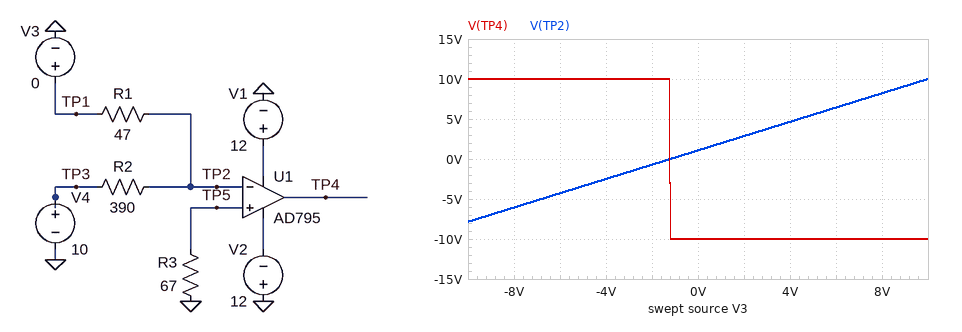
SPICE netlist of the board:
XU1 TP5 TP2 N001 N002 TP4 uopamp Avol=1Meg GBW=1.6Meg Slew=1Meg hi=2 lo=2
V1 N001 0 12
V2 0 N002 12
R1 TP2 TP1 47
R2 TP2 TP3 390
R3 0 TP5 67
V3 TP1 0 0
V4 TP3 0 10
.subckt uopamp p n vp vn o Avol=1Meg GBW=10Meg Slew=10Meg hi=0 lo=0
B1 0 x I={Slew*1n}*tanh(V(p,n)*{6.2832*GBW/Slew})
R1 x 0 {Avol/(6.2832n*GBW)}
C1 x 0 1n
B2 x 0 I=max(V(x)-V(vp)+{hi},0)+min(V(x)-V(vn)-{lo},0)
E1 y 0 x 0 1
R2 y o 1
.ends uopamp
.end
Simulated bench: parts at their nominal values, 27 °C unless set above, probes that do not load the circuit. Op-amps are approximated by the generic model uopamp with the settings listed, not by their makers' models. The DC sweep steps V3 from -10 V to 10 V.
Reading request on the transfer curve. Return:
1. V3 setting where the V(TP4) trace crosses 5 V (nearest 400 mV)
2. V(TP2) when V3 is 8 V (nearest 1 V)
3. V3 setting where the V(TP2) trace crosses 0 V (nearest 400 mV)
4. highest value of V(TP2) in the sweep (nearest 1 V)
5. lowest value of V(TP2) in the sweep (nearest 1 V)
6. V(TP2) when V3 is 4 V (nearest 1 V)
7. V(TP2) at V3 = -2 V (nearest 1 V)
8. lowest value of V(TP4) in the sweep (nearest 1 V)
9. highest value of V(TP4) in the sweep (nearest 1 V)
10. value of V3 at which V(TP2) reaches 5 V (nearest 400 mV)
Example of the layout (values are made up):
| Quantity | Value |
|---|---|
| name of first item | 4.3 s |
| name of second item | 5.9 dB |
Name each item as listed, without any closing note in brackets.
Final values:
| Quantity | Value |
|---|---|
| V3 setting where the V(TP4) trace crosses 5 V | -1.2 V |
| V(TP2) when V3 is 8 V | 8 V |
| V3 setting where the V(TP2) trace crosses 0 V | -1.2 V |
| highest value of V(TP2) in the sweep | 10 V |
| lowest value of V(TP2) in the sweep | -8 V |
| V(TP2) when V3 is 4 V | 5 V |
| V(TP2) at V3 = -2 V | -1 V |
| lowest value of V(TP4) in the sweep | -10 V |
| highest value of V(TP4) in the sweep | 10 V |
| value of V3 at which V(TP2) reaches 5 V | 4.4 V |
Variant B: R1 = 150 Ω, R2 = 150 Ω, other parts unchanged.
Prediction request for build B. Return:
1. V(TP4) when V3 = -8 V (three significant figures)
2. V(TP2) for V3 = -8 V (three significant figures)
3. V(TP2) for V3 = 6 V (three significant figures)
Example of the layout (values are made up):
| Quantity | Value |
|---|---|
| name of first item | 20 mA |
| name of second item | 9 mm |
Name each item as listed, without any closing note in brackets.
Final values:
| Quantity | Value |
|---|---|
| V(TP4) when V3 = -8 V | -10.0 V |
| V(TP2) for V3 = -8 V | 1.00 V |
| V(TP2) for V3 = 6 V | 8.00 V |
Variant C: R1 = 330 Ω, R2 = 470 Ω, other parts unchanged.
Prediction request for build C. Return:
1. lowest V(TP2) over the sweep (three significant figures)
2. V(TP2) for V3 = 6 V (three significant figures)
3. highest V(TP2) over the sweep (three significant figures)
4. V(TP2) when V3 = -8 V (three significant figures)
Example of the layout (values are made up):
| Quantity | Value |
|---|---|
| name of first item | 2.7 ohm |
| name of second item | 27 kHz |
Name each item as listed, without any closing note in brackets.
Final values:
| Quantity | Value |
|---|---|
| lowest V(TP2) over the sweep | -1.75 V |
| V(TP2) for V3 = 6 V | 7.65 V |
| highest V(TP2) over the sweep | 10.0 V |
| V(TP2) when V3 = -8 V | -575 mV |
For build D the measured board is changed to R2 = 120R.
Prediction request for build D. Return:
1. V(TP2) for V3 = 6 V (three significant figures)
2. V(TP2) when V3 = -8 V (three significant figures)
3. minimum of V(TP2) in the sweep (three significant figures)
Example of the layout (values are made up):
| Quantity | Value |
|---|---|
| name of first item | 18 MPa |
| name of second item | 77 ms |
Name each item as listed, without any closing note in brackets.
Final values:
| Quantity | Value |
|---|---|
| V(TP2) for V3 = 6 V | 7.13 V |
| V(TP2) when V3 = -8 V | -2.93 V |
| minimum of V(TP2) in the sweep | -4.37 V |
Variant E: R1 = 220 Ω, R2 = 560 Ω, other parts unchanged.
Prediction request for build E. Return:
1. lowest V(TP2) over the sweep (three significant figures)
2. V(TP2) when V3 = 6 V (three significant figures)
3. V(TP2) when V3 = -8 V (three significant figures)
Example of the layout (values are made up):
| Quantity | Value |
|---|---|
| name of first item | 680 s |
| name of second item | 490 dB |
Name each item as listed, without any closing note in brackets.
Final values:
| Quantity | Value |
|---|---|
| lowest V(TP2) over the sweep | -4.36 V |
| V(TP2) when V3 = 6 V | 7.13 V |
| V(TP2) when V3 = -8 V | -2.92 V |
